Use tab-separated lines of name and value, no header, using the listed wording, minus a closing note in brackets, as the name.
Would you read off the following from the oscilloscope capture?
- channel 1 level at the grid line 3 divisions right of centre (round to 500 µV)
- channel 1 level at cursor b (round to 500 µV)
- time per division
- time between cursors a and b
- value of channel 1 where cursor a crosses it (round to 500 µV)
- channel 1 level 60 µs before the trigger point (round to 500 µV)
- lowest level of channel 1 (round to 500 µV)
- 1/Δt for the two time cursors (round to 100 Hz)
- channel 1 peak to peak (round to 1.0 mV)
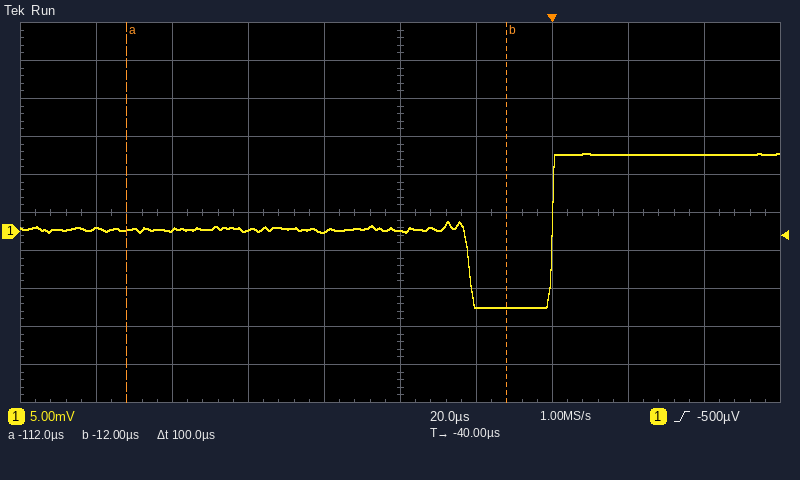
channel 1 level at the grid line 3 divisions right of centre	10.0 mV
channel 1 level at cursor b	-10.0 mV
time per division	20 µs
time between cursors a and b	100 µs
value of channel 1 where cursor a crosses it	0.0 mV
channel 1 level 60 µs before the trigger point	0.0 mV
lowest level of channel 1	-10.0 mV
1/Δt for the two time cursors	10.0 kHz
channel 1 peak to peak	20.0 mV
